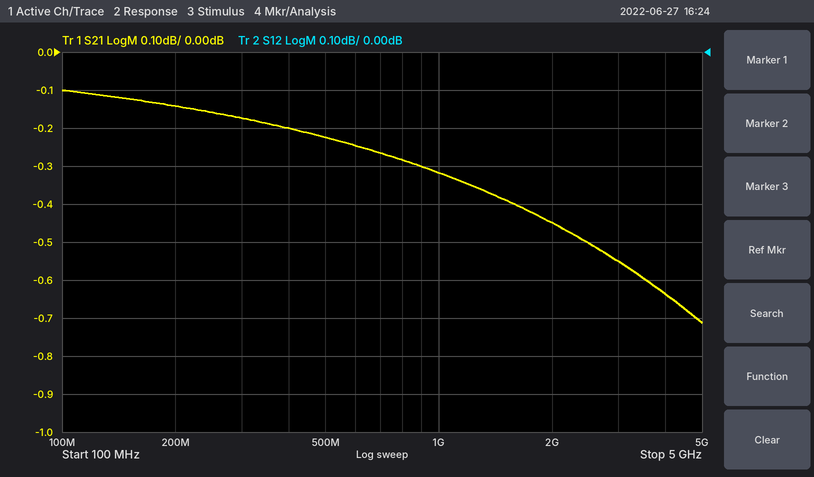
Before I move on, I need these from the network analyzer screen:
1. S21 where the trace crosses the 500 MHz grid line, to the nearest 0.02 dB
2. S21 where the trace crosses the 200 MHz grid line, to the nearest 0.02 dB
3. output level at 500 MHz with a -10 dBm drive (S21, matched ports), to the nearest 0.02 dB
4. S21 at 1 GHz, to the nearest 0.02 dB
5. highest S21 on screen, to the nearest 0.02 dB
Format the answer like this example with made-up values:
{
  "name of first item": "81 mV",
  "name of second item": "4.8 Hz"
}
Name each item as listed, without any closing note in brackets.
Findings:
{
  "S21 where the trace crosses the 500 MHz grid line, to the nearest 0.02 dB": "-0.22 dB",
  "S21 where the trace crosses the 200 MHz grid line, to the nearest 0.02 dB": "-0.14 dB",
  "output level at 500 MHz with a -10 dBm drive (S21, matched ports), to the nearest 0.02 dB": "-10.22 dBm",
  "S21 at 1 GHz, to the nearest 0.02 dB": "-0.32 dB",
  "highest S21 on screen, to the nearest 0.02 dB": "-0.10 dB"
}
